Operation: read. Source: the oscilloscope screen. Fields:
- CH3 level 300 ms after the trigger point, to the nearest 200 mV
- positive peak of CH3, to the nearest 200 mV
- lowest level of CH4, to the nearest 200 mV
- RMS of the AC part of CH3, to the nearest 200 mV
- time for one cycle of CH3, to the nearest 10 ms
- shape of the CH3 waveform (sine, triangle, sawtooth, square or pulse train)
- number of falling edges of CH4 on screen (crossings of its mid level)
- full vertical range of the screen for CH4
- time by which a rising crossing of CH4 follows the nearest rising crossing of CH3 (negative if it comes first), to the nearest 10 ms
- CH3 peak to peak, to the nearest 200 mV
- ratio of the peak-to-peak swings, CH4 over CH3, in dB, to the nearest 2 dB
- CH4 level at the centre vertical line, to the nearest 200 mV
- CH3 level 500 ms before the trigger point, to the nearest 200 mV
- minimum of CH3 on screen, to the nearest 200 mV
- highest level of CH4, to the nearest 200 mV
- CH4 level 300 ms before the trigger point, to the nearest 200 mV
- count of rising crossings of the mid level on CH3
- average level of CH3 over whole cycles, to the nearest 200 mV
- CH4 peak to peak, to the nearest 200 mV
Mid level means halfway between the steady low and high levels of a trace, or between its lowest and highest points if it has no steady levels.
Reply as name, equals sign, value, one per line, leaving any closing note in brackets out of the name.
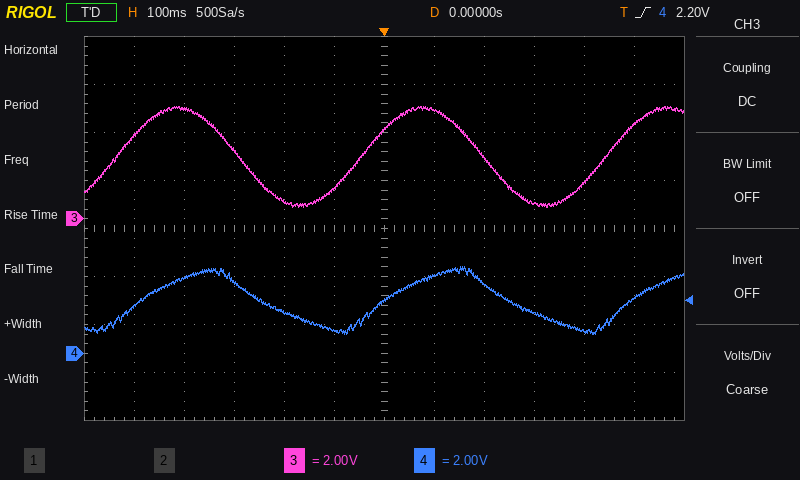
CH3 level 300 ms after the trigger point, to the nearest 200 mV = 600 mV
positive peak of CH3, to the nearest 200 mV = 4.6 V
lowest level of CH4, to the nearest 200 mV = 800 mV
RMS of the AC part of CH3, to the nearest 200 mV = 1.4 V
time for one cycle of CH3, to the nearest 10 ms = 490 ms
shape of the CH3 waveform = sine
number of falling edges of CH4 on screen = 2
full vertical range of the screen for CH4 = 16 V
time by which a rising crossing of CH4 follows the nearest rising crossing of CH3 (negative if it comes first), to the nearest 10 ms = +50 ms
CH3 peak to peak, to the nearest 200 mV = 4.2 V
ratio of the peak-to-peak swings, CH4 over CH3, in dB, to the nearest 2 dB = -4 dB
CH4 level at the centre vertical line, to the nearest 200 mV = 2.2 V
CH3 level 500 ms before the trigger point, to the nearest 200 mV = 3.4 V
minimum of CH3 on screen, to the nearest 200 mV = 400 mV
highest level of CH4, to the nearest 200 mV = 3.6 V
CH4 level 300 ms before the trigger point, to the nearest 200 mV = 3.0 V
count of rising crossings of the mid level on CH3 = 3
average level of CH3 over whole cycles, to the nearest 200 mV = 2.6 V
CH4 peak to peak, to the nearest 200 mV = 2.8 V
